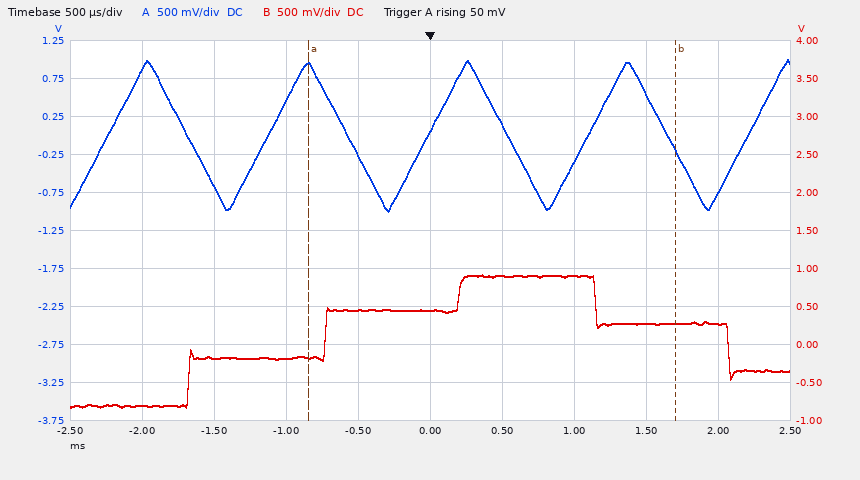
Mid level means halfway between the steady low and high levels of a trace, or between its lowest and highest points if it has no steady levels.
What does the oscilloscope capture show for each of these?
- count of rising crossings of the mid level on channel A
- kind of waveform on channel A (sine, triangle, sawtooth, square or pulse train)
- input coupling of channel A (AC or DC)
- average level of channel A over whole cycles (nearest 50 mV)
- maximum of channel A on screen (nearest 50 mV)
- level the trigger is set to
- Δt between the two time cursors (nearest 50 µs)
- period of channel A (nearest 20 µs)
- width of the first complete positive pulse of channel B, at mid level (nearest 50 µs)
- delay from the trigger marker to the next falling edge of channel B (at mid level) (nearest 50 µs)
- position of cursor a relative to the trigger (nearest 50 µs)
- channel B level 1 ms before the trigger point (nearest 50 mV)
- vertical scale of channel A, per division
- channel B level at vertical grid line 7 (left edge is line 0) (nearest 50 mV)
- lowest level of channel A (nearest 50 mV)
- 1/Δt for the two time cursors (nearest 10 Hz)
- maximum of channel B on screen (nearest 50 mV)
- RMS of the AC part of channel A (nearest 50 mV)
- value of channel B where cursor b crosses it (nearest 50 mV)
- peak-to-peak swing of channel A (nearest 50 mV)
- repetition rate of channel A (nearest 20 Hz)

5
triangle
DC
0 mV
1.00 V
50 mV
2.55 ms
1.12 ms
2.80 ms
2.05 ms
-850 µs
-200 mV
500 mV
900 mV
-1.00 V
390 Hz
900 mV
600 mV
300 mV
2.00 V
900 Hz
